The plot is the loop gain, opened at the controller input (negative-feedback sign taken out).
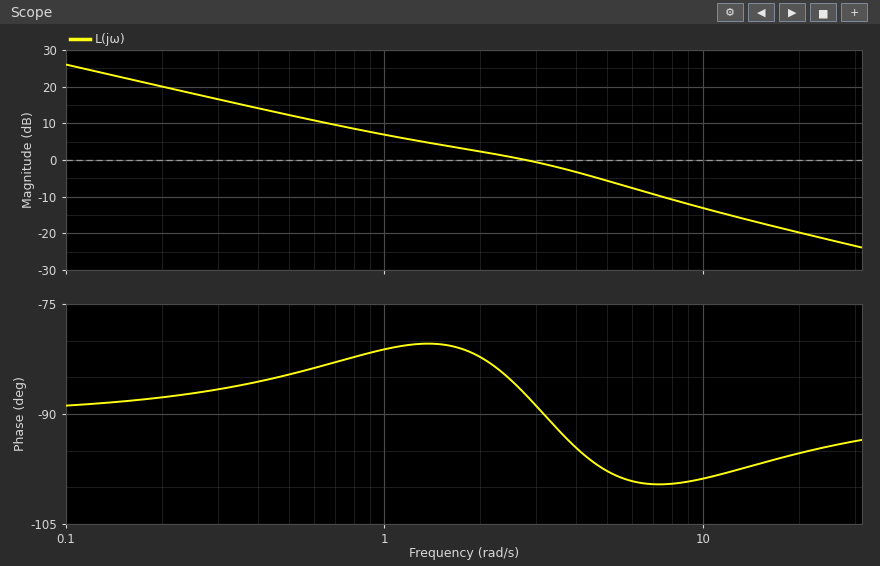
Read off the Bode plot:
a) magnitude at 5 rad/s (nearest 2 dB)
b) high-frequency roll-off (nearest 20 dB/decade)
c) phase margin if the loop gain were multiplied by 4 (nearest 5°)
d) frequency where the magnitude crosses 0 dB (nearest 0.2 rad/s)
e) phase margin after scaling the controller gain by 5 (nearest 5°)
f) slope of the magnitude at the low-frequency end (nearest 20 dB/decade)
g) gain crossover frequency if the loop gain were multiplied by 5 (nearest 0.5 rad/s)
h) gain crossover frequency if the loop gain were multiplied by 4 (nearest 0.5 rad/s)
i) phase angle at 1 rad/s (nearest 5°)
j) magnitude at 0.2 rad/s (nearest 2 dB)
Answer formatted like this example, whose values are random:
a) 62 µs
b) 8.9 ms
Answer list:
a) -6 dB
b) -20 dB/decade
c) 80°
d) 2.8 rad/s
e) 80°
f) -20 dB/decade
g) 11.0 rad/s
h) 9.0 rad/s
i) -80°
j) 20 dB
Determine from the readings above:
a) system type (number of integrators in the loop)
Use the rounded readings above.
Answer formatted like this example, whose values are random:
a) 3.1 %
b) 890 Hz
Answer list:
a) 1
